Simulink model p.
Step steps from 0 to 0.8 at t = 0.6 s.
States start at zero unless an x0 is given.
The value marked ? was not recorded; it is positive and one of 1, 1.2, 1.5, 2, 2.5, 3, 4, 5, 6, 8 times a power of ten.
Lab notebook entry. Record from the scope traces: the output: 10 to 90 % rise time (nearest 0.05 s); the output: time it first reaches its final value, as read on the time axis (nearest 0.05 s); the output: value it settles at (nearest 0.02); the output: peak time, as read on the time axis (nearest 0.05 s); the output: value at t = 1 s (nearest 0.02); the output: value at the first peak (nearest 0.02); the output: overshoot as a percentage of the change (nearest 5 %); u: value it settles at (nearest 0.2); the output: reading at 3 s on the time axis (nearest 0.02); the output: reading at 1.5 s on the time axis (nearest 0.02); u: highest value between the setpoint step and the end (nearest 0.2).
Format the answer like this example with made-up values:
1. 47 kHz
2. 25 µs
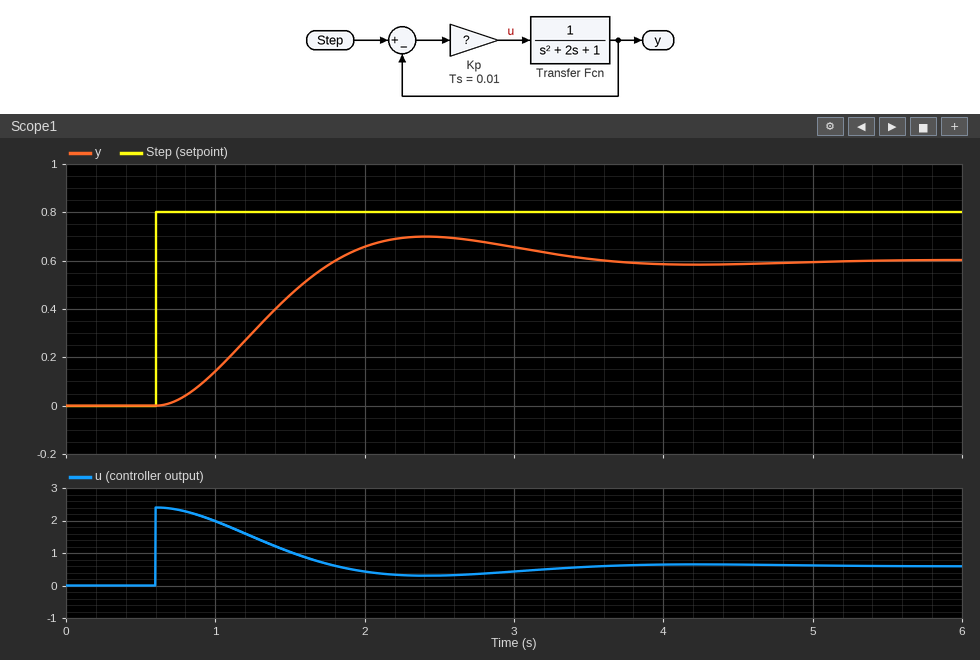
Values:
1. 0.80 s
2. 1.80 s
3. 0.60
4. 2.40 s
5. 0.14
6. 0.70
7. 15 %
8. 0.6
9. 0.66
10. 0.46
11. 2.4
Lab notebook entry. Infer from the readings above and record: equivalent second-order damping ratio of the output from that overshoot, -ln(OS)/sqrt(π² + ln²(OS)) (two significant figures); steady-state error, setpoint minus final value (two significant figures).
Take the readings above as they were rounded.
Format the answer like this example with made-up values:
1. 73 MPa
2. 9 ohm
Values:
1. 0.52
2. 0.20
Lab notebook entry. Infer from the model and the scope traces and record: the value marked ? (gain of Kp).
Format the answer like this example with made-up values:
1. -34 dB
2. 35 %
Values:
1. 3
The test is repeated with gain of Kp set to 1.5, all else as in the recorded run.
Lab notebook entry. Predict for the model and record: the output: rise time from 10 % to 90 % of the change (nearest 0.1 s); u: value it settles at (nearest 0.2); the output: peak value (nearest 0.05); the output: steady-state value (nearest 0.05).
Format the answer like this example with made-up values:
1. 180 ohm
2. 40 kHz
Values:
1. 1.2 s
2. 0.4
3. 0.50
4. 0.50
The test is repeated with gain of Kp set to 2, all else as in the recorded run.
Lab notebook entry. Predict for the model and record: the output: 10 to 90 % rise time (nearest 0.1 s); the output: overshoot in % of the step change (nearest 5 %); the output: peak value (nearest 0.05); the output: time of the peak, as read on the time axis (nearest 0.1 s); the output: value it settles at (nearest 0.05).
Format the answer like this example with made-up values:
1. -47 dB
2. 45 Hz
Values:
1. 1.0 s
2. 10 %
3. 0.60
4. 2.8 s
5. 0.55
